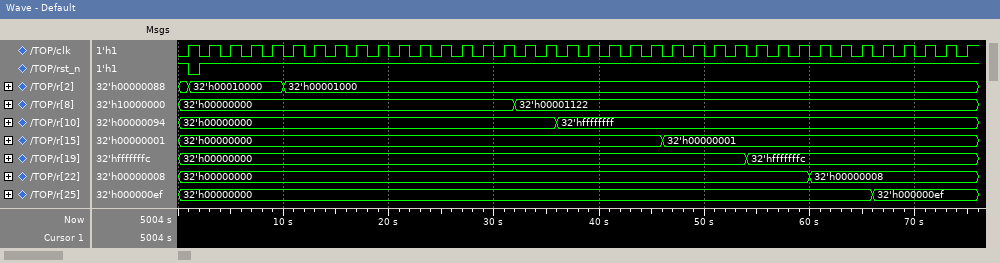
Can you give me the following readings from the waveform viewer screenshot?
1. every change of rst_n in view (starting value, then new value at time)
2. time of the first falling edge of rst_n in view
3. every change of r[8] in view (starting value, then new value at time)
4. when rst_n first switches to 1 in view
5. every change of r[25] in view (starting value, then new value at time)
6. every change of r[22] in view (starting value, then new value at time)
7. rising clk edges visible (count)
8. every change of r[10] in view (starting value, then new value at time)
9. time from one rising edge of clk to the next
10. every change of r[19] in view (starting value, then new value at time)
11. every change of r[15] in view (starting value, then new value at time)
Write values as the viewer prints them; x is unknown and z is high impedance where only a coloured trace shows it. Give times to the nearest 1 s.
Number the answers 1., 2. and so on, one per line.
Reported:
1. 1, 0 at 1 s, 1 at 2 s
2. 1 s
3. 32'h00000000, 32'h00001122 at 32 s
4. 2 s
5. 32'h00000000, 32'h000000ef at 66 s
6. 32'h00000000, 32'h00000008 at 60 s
7. 38
8. 32'h00000000, 32'hffffffff at 36 s
9. 2 s
10. 32'h00000000, 32'hfffffffc at 54 s
11. 32'h00000000, 32'h00000001 at 46 s
